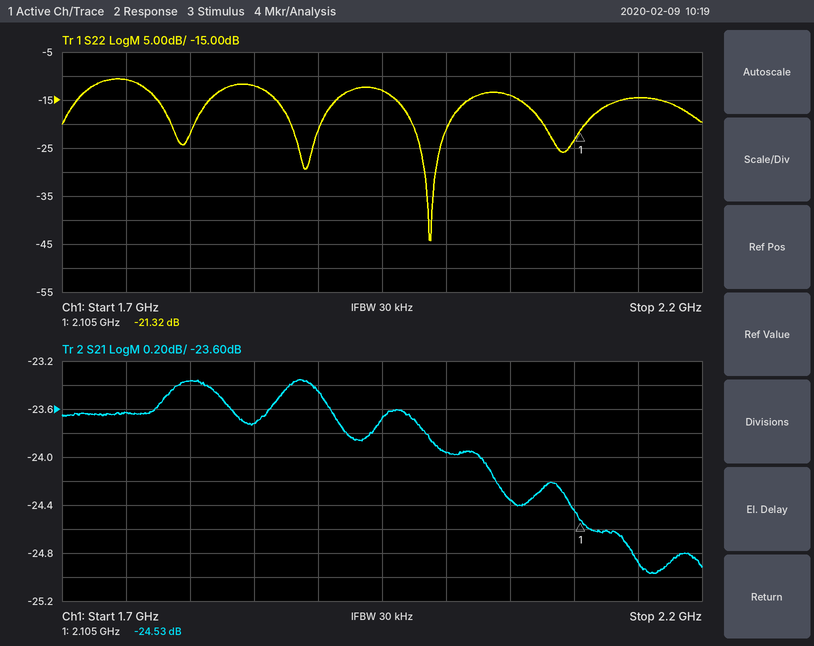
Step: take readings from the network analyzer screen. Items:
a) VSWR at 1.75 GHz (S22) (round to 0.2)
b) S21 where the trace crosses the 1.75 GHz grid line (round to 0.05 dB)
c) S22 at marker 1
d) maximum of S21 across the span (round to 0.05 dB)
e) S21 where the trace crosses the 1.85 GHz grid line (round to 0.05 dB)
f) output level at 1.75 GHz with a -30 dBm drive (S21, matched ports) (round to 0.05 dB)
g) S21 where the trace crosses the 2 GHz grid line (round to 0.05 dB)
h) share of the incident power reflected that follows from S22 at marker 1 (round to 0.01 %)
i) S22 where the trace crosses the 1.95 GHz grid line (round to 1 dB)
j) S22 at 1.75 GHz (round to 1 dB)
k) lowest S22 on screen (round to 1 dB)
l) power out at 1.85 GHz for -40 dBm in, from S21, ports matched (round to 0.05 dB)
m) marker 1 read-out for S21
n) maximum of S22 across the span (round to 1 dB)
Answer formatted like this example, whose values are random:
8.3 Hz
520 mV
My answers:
1.8
-23.65 dB
-21.32 dB
-23.35 dB
-23.70 dB
-53.65 dBm
-23.95 dB
0.74 %
-13 dB
-11 dB
-44 dB
-63.70 dBm
-24.53 dB
-11 dB
